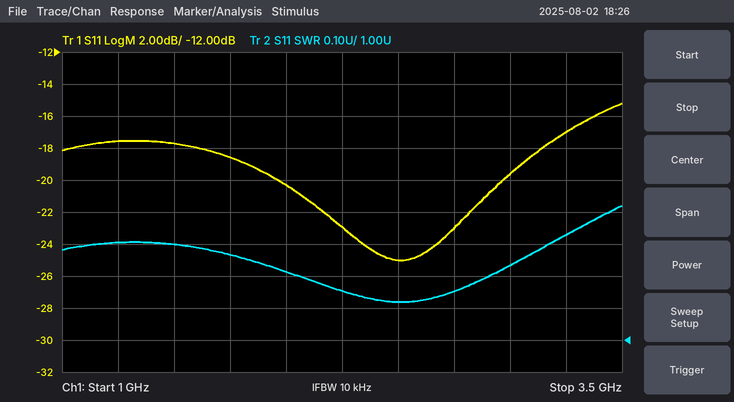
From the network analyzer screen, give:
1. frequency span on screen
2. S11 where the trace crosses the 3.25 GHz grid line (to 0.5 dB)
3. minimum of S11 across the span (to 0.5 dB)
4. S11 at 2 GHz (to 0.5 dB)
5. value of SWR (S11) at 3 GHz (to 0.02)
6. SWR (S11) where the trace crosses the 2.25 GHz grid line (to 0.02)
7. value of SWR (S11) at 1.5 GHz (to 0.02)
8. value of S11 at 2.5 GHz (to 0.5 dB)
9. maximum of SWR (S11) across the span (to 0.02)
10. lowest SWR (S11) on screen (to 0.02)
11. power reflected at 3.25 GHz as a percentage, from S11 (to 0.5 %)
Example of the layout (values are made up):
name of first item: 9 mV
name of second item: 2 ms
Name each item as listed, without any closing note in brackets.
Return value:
frequency span on screen: 2.5 GHz
S11 where the trace crosses the 3.25 GHz grid line: -17.0 dB
minimum of S11 across the span: -25.0 dB
S11 at 2 GHz: -20.5 dB
value of SWR (S11) at 3 GHz: 1.24
SWR (S11) where the trace crosses the 2.25 GHz grid line: 1.16
value of SWR (S11) at 1.5 GHz: 1.30
value of S11 at 2.5 GHz: -25.0 dB
maximum of SWR (S11) across the span: 1.42
lowest SWR (S11) on screen: 1.12
power reflected at 3.25 GHz as a percentage, from S11: 2.0 %
